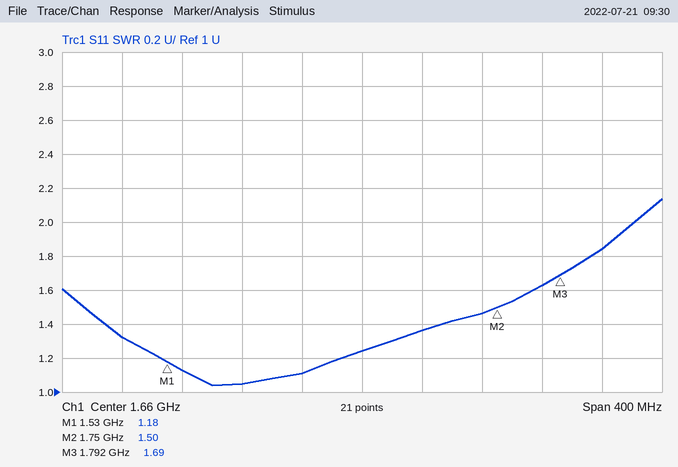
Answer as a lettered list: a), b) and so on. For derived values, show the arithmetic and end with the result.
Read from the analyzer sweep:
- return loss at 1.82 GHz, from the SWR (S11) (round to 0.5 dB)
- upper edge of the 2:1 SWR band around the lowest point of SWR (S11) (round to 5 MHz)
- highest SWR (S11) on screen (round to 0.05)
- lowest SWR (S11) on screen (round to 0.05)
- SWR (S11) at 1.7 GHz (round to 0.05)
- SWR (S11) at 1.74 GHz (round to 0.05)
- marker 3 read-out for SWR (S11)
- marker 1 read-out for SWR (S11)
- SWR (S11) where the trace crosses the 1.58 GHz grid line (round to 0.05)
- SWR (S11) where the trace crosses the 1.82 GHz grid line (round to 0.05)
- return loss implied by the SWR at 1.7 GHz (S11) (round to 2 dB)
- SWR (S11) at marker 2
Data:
a) −20 log10((1.85 − 1)/(1.85 + 1)) ≈ 10.5 dB
b) 1.840 GHz
c) 2.15
d) 1.05
e) 1.35
f) 1.45
g) 1.69
h) 1.18
i) 1.05
j) 1.85
k) −20 log10((1.35 − 1)/(1.35 + 1)) ≈ 16 dB
l) 1.50
